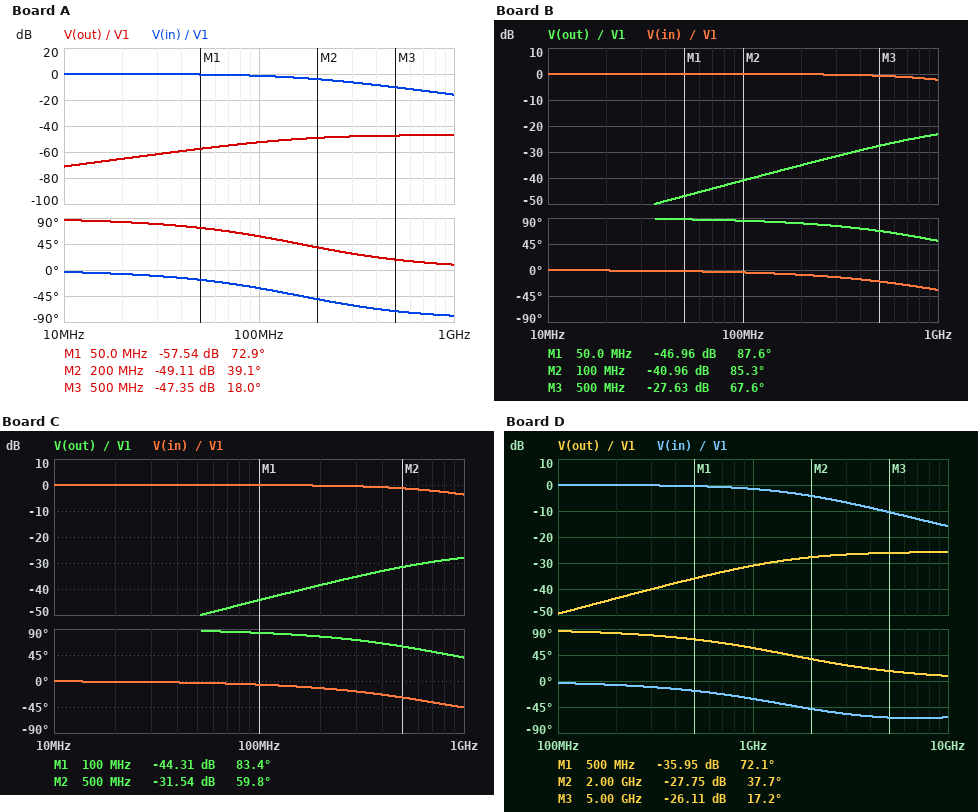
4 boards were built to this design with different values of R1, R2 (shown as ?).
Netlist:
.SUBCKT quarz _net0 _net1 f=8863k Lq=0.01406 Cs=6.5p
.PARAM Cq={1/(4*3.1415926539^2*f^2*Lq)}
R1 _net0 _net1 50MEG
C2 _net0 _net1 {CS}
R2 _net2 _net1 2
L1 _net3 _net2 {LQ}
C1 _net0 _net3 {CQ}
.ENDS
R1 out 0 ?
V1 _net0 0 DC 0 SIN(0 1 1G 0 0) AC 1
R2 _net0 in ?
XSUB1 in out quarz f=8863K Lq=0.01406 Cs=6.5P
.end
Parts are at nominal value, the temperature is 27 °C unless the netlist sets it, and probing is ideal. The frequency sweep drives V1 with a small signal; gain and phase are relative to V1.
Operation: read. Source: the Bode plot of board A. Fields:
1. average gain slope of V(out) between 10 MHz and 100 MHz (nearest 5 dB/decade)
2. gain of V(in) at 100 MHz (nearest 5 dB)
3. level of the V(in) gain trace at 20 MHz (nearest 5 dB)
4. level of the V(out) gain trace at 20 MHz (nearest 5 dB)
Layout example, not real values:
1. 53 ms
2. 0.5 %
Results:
1. 20 dB/decade
2. 0 dB
3. 0 dB
4. -65 dB
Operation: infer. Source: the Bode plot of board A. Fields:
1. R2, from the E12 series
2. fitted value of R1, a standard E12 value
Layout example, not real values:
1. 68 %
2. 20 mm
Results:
1. 150 Ω
2. 0.68 Ω
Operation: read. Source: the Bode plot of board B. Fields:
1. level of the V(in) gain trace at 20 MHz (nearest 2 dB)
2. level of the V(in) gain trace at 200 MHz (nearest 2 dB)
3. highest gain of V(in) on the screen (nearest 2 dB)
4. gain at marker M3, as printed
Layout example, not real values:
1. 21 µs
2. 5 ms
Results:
1. 0 dB
2. 0 dB
3. 0 dB
4. -27.63 dB
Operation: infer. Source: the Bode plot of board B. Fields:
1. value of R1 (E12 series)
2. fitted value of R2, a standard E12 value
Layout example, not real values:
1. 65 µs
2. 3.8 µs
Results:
1. 2.2 Ω
2. 18 Ω
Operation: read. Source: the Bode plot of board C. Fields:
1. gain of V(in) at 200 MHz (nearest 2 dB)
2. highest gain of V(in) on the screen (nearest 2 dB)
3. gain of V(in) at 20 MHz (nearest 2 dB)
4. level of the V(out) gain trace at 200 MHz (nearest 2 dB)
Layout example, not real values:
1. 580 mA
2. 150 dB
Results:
1. 0 dB
2. 0 dB
3. 0 dB
4. -38 dB
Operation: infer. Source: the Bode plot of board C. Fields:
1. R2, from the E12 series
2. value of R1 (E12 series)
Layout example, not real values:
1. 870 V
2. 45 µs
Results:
1. 27 Ω
2. 1.5 Ω
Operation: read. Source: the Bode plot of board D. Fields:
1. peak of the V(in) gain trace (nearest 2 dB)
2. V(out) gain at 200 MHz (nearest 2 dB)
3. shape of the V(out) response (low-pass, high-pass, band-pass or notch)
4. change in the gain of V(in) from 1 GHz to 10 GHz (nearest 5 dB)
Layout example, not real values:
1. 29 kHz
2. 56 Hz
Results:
1. 0 dB
2. -44 dB
3. high-pass
4. -15 dB
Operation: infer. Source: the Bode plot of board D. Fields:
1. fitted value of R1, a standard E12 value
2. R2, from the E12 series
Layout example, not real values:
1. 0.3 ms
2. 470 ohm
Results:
1. 0.82 Ω
2. 15 Ω
